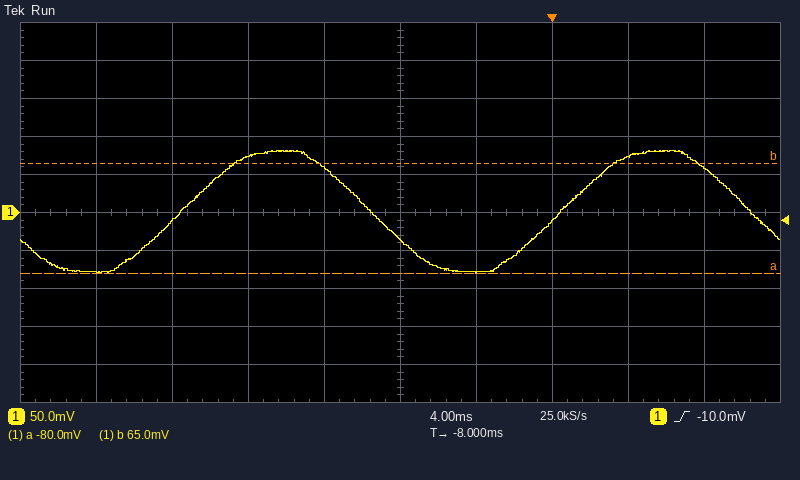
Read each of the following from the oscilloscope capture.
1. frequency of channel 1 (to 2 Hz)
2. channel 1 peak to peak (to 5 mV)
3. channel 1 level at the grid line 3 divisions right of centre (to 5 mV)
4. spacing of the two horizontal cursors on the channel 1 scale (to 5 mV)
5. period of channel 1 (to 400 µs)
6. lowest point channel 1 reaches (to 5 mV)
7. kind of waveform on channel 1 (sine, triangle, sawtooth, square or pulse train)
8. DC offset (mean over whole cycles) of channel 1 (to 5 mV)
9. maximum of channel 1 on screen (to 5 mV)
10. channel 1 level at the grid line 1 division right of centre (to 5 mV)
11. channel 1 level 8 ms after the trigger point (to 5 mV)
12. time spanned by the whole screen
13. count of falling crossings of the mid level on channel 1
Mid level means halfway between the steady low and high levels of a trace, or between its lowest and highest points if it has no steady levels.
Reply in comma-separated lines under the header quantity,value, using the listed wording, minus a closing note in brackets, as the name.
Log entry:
quantity,value
frequency of channel 1,50 Hz
channel 1 peak to peak,160 mV
channel 1 level at the grid line 3 divisions right of centre,75 mV
spacing of the two horizontal cursors on the channel 1 scale,145 mV
period of channel 1,20.0 ms
lowest point channel 1 reaches,-80 mV
kind of waveform on channel 1,sine
DC offset (mean over whole cycles) of channel 1,0 mV
maximum of channel 1 on screen,80 mV
channel 1 level at the grid line 1 division right of centre,-80 mV
channel 1 level 8 ms after the trigger point,60 mV
time spanned by the whole screen,40 ms
count of falling crossings of the mid level on channel 1,2
